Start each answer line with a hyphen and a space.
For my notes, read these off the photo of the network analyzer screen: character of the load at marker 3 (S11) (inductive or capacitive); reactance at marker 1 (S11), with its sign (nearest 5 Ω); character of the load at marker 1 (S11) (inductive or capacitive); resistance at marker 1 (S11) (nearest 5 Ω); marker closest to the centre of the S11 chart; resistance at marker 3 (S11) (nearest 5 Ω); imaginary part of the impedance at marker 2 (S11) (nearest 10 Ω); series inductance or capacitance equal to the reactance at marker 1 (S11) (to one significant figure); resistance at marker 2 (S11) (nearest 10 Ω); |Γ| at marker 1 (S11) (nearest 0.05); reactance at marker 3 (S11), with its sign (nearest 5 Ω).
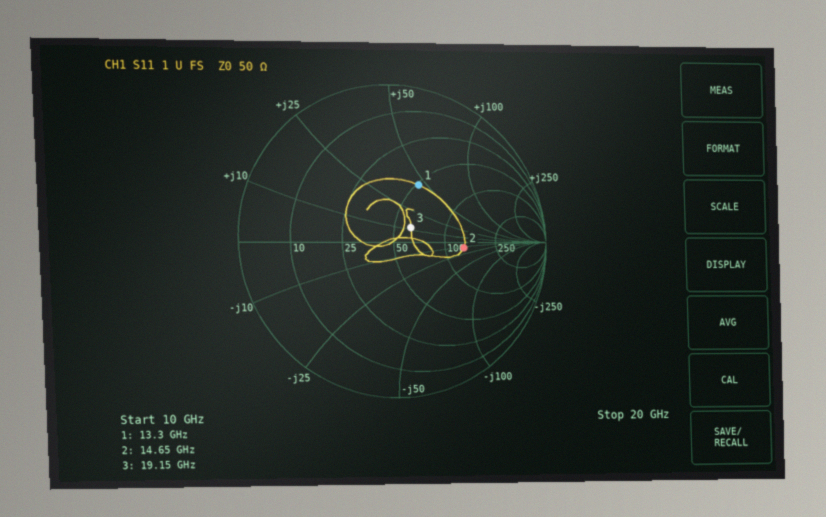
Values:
- inductive
- +45 Ω
- inductive
- 50 Ω
- marker 3
- 60 Ω
- -10 Ω
- 500 pH
- 130 Ω
- 0.40
- +10 Ω
